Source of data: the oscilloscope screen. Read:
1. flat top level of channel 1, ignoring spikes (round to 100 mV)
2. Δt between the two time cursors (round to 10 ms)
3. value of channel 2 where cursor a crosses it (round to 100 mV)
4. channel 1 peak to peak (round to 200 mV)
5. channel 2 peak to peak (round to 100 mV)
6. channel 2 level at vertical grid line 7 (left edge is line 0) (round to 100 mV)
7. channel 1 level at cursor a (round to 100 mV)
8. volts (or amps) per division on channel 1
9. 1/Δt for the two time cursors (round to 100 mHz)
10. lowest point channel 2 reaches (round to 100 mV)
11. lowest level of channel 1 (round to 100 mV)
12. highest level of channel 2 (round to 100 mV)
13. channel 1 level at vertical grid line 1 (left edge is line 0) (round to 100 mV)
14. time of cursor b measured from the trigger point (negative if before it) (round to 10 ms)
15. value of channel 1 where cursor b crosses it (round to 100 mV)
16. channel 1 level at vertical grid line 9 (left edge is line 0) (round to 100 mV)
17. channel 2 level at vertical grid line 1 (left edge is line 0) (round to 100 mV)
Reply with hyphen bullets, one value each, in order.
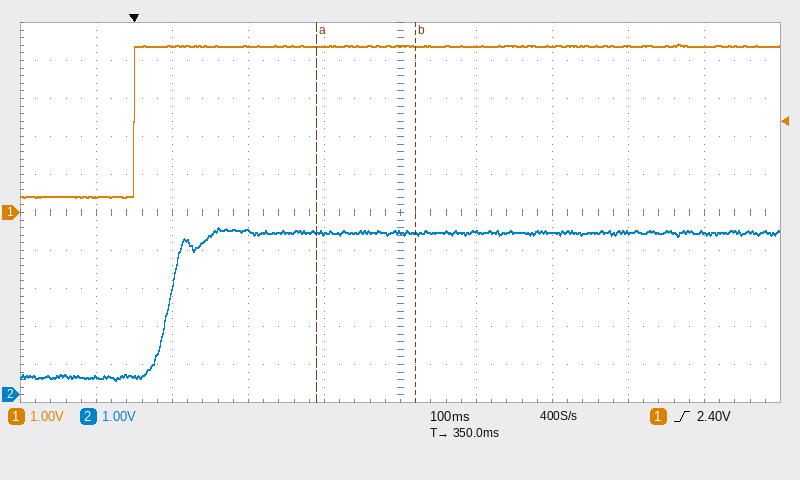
- 4.4 V
- 130 ms
- 4.3 V
- 4.0 V
- 4.0 V
- 4.3 V
- 4.4 V
- 1 V
- 7.7 Hz
- 400 mV
- 400 mV
- 4.4 V
- 400 mV
- +370 ms
- 4.4 V
- 4.4 V
- 500 mV
